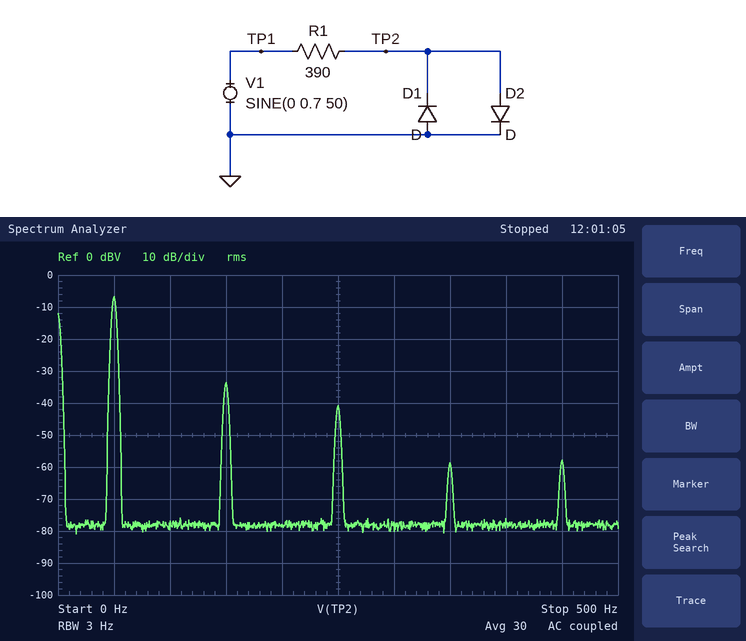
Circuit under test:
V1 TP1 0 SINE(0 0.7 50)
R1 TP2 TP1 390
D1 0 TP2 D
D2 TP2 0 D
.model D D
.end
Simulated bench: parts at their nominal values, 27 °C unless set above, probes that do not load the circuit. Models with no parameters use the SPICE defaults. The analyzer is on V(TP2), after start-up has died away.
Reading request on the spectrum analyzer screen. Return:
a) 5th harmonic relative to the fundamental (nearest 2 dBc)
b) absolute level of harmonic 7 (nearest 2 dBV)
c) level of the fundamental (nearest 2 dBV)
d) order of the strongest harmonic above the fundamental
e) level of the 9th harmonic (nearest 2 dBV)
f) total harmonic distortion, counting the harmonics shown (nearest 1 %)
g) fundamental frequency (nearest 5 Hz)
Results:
-34 dBc
-58 dBV
-6 dBV
3
-58 dBV
5 %
50 Hz
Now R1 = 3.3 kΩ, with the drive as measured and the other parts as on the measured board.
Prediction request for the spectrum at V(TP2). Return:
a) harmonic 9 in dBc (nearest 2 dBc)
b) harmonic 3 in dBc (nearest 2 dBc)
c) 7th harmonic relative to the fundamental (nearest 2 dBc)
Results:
-46 dBc
-22 dBc
-48 dBc
